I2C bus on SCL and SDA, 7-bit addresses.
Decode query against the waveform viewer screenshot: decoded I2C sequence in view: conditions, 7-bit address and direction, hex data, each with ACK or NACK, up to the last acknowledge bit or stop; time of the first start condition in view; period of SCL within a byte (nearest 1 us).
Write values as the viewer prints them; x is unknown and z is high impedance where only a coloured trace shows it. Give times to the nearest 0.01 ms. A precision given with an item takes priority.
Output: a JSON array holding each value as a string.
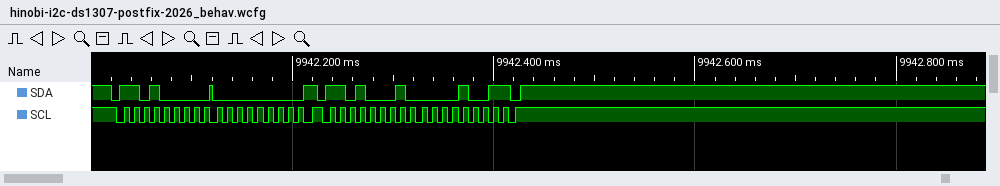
["start, address 68 write ACK, 00 ACK, repeated start, address 68 read ACK, 09 NACK, stop", "9942.02 ms", "10 us"]
